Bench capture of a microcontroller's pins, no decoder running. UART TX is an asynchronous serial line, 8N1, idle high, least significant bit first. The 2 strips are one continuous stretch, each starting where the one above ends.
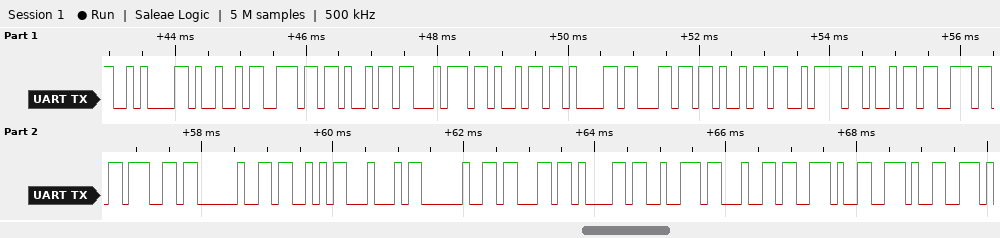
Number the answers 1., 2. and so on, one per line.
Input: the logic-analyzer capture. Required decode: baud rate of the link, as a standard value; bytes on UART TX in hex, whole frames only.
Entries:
1. 9600 baud
2. 0A 49 6E 69 74 69 61 6C 69 7A 69 6E 67 20 53 44 20 63 61 72 64 2E 2E
